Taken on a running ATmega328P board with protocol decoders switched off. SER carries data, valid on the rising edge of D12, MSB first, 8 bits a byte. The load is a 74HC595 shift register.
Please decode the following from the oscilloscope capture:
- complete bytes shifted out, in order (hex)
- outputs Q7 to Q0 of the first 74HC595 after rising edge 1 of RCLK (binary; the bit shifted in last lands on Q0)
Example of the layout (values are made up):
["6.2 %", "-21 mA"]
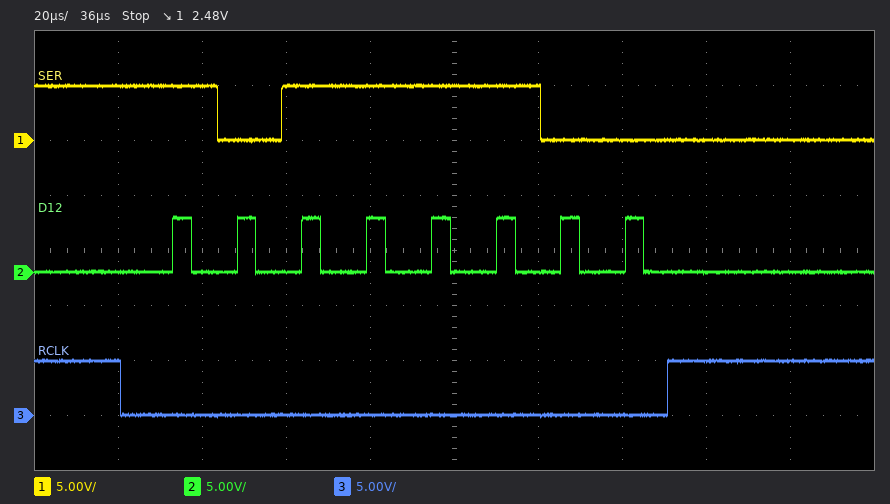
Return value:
["BC", "10111100"]
